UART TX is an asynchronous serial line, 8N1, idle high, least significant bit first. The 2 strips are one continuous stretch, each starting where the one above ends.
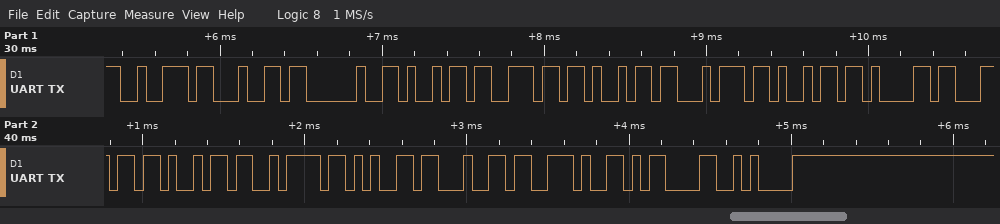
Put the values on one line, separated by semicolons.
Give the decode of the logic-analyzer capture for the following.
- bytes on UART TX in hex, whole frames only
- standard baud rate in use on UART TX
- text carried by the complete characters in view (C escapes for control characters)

72 64 20 69 6E 69 74 69 61 6C 69 7A 65 64 2E 0D 0A; 19200 baud; "rd initialized.\r\n"
